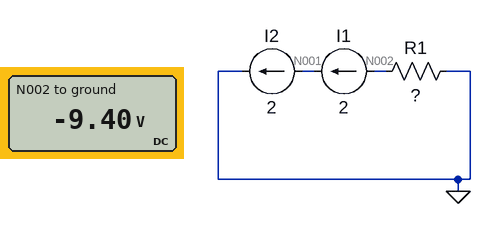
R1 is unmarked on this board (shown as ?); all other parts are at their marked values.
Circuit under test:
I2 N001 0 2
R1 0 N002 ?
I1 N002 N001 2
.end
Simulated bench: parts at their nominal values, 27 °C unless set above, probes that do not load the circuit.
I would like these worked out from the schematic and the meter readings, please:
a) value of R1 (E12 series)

4.7 Ω
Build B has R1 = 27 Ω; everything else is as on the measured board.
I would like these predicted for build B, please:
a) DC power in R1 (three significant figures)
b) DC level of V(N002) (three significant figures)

108 W
-54.0 V
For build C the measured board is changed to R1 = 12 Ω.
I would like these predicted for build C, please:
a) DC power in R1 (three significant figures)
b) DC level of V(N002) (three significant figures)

48.0 W
-24.0 V
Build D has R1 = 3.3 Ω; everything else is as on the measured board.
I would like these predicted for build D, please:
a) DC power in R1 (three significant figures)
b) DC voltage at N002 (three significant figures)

13.2 W
-6.60 V
